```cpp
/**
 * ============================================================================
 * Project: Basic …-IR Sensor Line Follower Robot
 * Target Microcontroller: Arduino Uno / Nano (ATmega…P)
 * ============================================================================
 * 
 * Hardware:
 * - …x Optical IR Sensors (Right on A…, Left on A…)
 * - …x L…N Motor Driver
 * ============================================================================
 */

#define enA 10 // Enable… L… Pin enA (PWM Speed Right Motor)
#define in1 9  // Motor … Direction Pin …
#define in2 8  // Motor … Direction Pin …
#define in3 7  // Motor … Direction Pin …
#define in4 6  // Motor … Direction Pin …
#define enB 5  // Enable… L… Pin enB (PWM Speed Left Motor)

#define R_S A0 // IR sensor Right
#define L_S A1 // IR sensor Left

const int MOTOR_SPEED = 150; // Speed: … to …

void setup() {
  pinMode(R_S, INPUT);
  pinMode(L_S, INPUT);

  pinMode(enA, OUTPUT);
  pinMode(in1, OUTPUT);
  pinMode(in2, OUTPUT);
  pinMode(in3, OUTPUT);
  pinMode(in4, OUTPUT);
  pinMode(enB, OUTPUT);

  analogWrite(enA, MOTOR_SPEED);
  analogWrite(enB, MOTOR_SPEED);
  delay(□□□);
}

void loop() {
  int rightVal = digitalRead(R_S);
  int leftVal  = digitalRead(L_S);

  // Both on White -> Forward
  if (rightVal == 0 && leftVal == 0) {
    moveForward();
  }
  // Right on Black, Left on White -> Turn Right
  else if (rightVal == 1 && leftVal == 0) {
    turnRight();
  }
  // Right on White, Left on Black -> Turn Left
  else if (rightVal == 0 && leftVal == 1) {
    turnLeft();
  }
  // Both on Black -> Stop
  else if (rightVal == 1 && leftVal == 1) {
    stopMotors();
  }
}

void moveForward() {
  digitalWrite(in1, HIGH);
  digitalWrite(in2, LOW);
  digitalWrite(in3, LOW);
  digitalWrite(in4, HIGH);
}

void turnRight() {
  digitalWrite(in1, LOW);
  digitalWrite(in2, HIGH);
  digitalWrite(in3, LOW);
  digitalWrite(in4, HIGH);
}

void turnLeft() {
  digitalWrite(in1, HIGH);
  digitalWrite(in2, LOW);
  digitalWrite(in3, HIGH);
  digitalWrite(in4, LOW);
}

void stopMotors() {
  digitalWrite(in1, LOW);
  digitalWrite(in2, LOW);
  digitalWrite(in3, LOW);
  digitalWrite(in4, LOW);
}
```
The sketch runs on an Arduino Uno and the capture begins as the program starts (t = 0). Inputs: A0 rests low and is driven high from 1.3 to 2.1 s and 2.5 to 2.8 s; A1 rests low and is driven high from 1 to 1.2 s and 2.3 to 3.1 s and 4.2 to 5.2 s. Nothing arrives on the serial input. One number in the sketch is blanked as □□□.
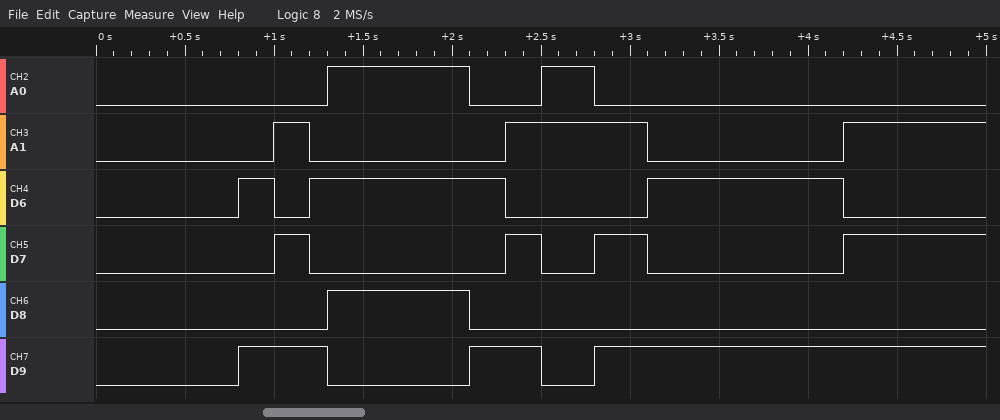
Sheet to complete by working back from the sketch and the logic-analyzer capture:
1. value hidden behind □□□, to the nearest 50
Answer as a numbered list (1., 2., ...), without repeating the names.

1. 800
